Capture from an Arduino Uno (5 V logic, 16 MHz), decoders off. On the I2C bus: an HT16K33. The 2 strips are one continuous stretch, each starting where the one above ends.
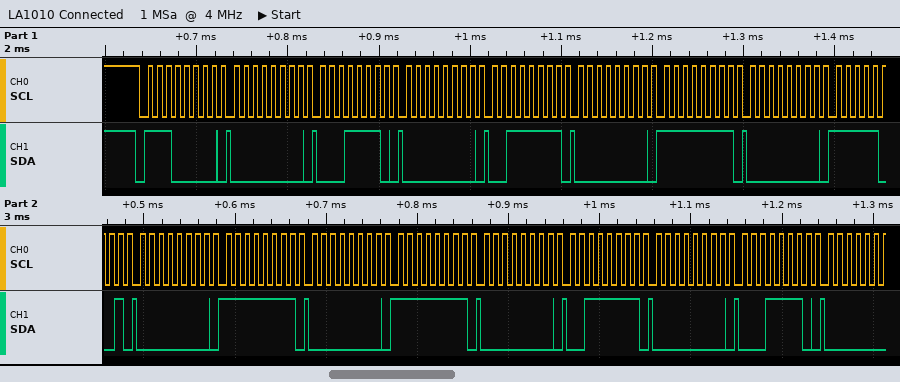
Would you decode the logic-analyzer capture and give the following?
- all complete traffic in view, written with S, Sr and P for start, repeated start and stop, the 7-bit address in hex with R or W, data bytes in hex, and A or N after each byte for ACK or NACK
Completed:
S 70W A 00 A 1E A 00 A 3F A 00 A FF A 00 A F9 A 00 A FF A 00 A FF A 00 A 3F A 00 A 1E A
